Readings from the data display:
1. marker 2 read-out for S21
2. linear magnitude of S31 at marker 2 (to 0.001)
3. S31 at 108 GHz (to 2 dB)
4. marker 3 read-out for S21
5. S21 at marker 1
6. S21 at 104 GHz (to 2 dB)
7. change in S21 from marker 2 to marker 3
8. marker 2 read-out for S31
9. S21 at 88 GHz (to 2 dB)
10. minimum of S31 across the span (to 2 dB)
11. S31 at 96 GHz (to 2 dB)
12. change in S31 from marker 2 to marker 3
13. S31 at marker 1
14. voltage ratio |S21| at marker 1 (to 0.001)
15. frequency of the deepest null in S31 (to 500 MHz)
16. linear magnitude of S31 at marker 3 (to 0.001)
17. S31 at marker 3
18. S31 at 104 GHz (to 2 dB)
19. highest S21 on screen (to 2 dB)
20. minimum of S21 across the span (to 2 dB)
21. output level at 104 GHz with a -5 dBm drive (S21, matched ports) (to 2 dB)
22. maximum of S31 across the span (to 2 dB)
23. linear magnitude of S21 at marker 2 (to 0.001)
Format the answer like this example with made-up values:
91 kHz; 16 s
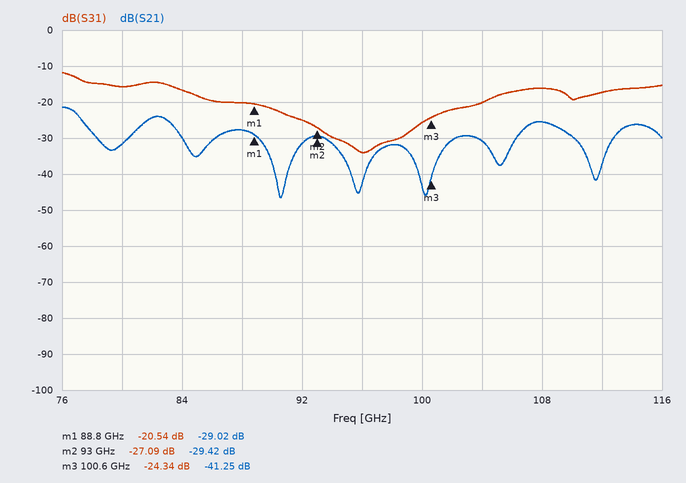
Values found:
-29.42 dB; 0.044; -16 dB; -41.25 dB; -29.02 dB; -30 dB; -11.83 dB; -27.09 dB; -28 dB; -34 dB; -34 dB; 2.75 dB; -20.54 dB; 0.035; 96.0 GHz; 0.061; -24.34 dB; -20 dB; -22 dB; -46 dB; -36 dBm; -12 dB; 0.034
